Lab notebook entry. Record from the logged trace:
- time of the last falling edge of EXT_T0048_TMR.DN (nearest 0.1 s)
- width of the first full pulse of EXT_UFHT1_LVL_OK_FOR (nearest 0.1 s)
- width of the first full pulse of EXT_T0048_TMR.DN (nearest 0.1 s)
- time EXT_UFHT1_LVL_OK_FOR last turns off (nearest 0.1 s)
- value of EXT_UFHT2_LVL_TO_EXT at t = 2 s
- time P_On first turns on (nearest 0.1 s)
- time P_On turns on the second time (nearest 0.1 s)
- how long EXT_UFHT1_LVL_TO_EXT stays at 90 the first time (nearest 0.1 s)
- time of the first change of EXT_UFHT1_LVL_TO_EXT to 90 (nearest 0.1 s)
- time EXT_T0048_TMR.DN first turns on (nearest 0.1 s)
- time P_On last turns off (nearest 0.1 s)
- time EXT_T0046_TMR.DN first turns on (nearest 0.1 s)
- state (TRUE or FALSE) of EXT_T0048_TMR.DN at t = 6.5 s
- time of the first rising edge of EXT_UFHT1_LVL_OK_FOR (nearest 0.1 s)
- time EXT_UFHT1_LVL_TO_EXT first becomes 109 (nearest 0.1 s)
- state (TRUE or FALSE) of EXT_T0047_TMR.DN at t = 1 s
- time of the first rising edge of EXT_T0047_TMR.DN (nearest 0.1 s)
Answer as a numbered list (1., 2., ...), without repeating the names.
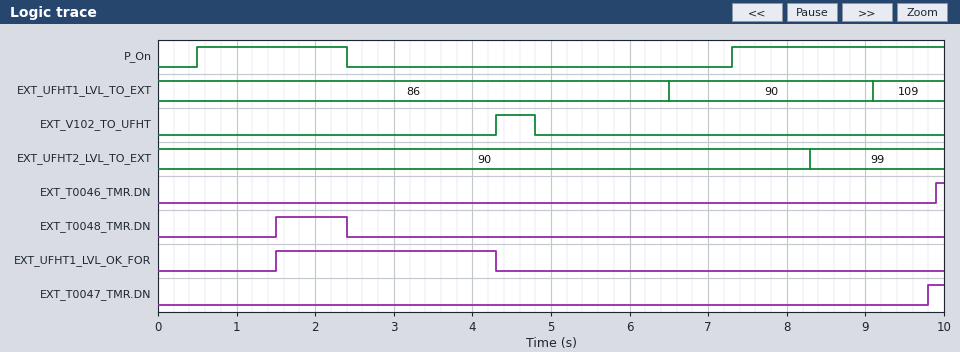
1. 2.4 s
2. 2.8 s
3. 0.9 s
4. 4.3 s
5. 90
6. 0.5 s
7. 7.3 s
8. 2.6 s
9. 6.5 s
10. 1.5 s
11. 2.4 s
12. 9.9 s
13. FALSE
14. 1.5 s
15. 9.1 s
16. FALSE
17. 9.8 s
